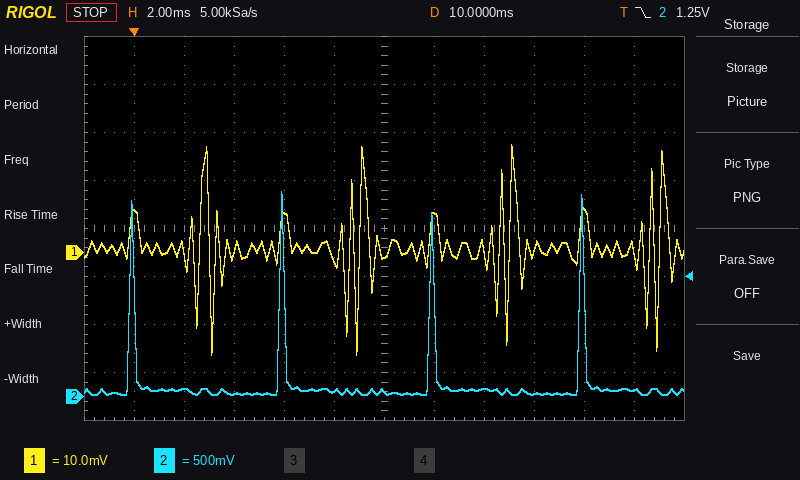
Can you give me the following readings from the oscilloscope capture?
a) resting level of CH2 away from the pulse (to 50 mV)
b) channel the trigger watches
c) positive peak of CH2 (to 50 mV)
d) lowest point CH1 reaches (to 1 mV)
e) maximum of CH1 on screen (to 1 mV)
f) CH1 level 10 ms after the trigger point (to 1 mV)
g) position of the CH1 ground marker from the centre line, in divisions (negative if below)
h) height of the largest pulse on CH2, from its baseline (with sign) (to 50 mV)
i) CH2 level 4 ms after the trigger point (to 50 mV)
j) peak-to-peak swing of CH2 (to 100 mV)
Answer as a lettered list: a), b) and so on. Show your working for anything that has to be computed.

a) 50 mV
b) CH2
c) 2.15 V
d) -21 mV
e) 22 mV
f) -1 mV
g) -0.5 div
h) 2.15 V − (50 mV) = +2.10 V
i) 50 mV
j) 2.10 V
